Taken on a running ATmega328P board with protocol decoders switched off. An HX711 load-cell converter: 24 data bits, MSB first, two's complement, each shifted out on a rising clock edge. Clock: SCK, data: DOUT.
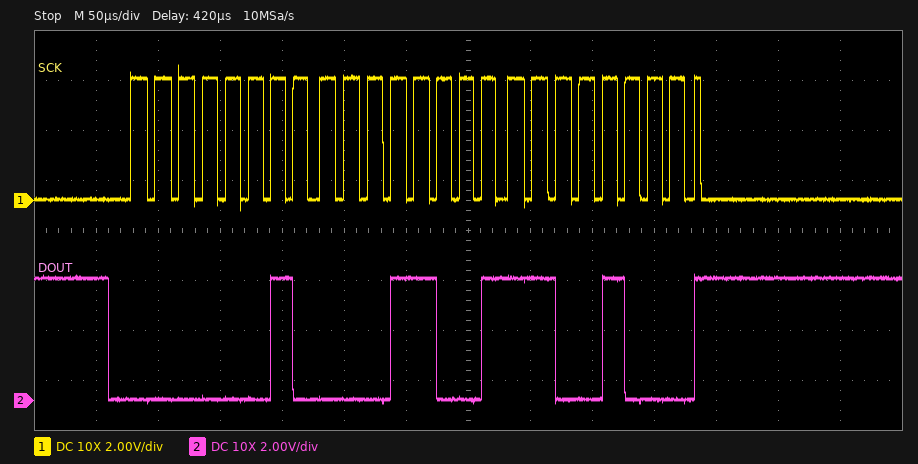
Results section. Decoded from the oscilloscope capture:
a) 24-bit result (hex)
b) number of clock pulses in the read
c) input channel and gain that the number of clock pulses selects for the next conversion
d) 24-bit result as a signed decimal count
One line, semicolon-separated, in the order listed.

0x0219C8; 25; channel A, gain 128; 137672
